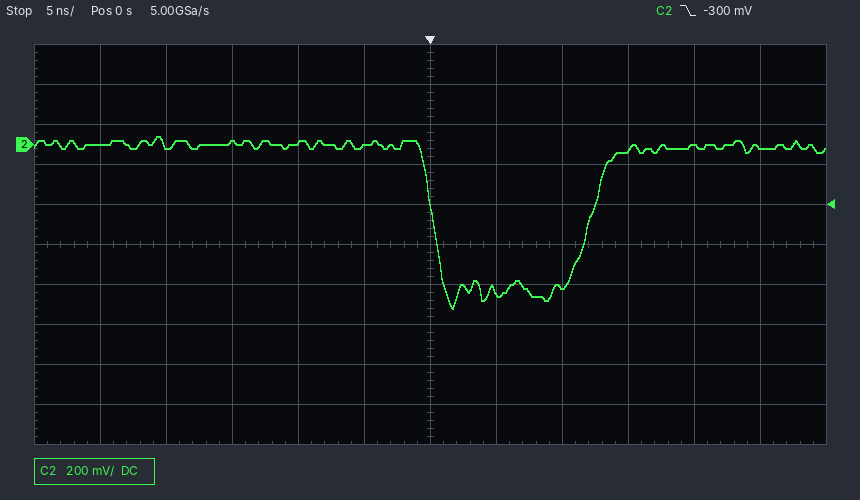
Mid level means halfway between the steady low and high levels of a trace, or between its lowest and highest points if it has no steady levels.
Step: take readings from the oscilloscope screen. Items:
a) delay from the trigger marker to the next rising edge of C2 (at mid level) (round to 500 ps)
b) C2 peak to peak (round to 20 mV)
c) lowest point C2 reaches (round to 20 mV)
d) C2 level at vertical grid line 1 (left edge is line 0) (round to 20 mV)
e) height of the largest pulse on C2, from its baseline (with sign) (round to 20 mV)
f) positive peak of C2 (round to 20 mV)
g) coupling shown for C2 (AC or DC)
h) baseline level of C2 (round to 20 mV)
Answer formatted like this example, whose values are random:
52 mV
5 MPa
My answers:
12.0 ns
860 mV
-820 mV
0 mV
-820 mV
40 mV
DC
0 mV
